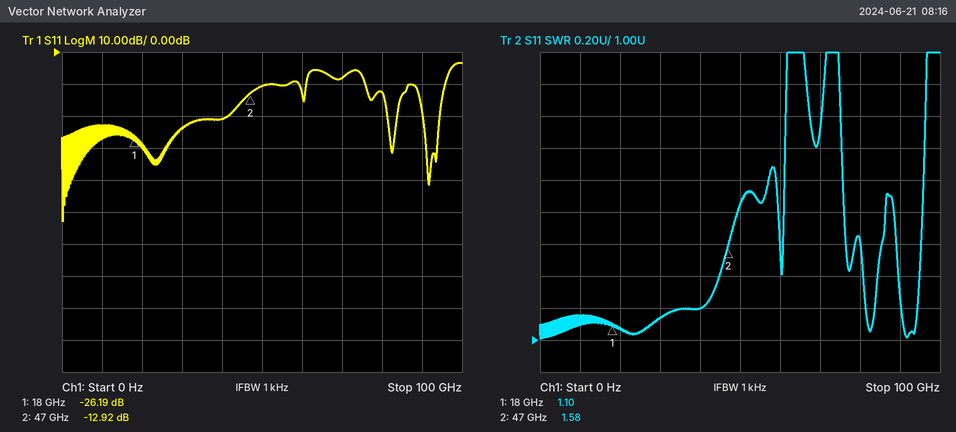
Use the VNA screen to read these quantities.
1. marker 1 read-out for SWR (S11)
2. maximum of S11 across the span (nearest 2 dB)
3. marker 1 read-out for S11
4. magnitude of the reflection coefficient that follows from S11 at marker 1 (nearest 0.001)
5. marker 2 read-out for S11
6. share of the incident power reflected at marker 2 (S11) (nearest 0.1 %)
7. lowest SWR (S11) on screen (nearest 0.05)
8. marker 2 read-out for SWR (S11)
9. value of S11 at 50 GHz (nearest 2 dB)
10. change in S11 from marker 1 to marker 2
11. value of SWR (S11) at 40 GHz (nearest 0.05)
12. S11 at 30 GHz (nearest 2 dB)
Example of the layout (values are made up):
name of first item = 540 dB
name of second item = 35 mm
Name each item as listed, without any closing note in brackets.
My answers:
marker 1 read-out for SWR = 1.10
maximum of S11 across the span = -4 dB
marker 1 read-out for S11 = -26.19 dB
magnitude of the reflection coefficient that follows from S11 at marker 1 = 0.049
marker 2 read-out for S11 = -12.92 dB
share of the incident power reflected at marker 2 (S11) = 5.1 %
lowest SWR (S11) on screen = 1.00
marker 2 read-out for SWR = 1.58
value of S11 at 50 GHz = -10 dB
change in S11 from marker 1 to marker 2 = 13.27 dB
value of SWR (S11) at 40 GHz = 1.20
S11 at 30 GHz = -24 dB
